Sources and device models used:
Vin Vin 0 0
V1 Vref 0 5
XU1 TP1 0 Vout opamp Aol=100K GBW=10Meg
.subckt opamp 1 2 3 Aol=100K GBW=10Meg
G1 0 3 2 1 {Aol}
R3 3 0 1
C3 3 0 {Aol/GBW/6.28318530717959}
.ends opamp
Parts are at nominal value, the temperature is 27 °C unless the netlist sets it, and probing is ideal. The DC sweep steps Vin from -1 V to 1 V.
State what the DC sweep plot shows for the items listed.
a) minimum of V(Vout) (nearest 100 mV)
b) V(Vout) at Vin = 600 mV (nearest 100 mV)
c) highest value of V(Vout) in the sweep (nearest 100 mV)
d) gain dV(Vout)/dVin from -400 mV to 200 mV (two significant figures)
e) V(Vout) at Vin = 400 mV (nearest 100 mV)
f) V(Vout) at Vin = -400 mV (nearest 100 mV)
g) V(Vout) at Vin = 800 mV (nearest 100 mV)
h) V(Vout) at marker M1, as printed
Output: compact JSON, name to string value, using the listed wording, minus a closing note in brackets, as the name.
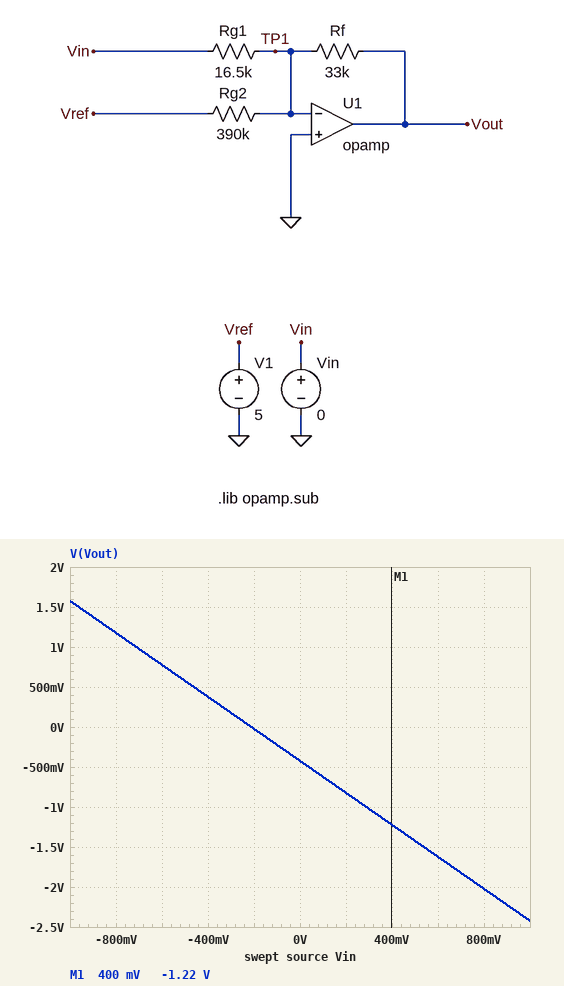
{"minimum of V(Vout)": "-2.4 V", "V(Vout) at Vin = 600 mV": "-1.6 V", "highest value of V(Vout) in the sweep": "1.6 V", "gain dV(Vout)/dVin from -400 mV to 200 mV": "-2.0 V/V", "V(Vout) at Vin = 400 mV": "-1.2 V", "V(Vout) at Vin = -400 mV": "400 mV", "V(Vout) at Vin = 800 mV": "-2.0 V", "V(Vout) at marker M1, as printed": "-1.22 V"}
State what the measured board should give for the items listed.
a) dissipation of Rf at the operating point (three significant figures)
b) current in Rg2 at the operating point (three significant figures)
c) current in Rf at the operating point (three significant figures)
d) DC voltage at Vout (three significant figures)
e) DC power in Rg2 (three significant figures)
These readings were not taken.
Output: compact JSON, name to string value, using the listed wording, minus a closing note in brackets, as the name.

{"dissipation of Rf at the operating point": "5.42 µW", "current in Rg2 at the operating point": "12.8 µA", "current in Rf at the operating point": "12.8 µA", "DC voltage at Vout": "-423 mV", "DC power in Rg2": "64.1 µW"}
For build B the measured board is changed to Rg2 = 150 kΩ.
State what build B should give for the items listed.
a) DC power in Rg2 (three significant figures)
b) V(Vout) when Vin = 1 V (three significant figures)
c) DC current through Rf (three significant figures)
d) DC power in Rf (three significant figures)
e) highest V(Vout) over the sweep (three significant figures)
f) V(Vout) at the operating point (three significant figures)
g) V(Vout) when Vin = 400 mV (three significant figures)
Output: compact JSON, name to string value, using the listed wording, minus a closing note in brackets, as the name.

{"DC power in Rg2": "167 µW", "V(Vout) when Vin = 1 V": "-3.10 V", "DC current through Rf": "33.3 µA", "DC power in Rf": "36.7 µW", "highest V(Vout) over the sweep": "900 mV", "V(Vout) at the operating point": "-1.10 V", "V(Vout) when Vin = 400 mV": "-1.90 V"}
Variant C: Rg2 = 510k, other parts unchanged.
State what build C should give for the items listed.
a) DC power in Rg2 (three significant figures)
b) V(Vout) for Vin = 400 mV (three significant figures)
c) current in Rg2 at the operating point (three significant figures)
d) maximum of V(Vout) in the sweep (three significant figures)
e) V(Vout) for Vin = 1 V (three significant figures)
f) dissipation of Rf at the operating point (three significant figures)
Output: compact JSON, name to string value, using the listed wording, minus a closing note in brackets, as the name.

{"DC power in Rg2": "49.0 µW", "V(Vout) for Vin = 400 mV": "-1.12 V", "current in Rg2 at the operating point": "9.80 µA", "maximum of V(Vout) in the sweep": "1.68 V", "V(Vout) for Vin = 1 V": "-2.32 V", "dissipation of Rf at the operating point": "3.17 µW"}
